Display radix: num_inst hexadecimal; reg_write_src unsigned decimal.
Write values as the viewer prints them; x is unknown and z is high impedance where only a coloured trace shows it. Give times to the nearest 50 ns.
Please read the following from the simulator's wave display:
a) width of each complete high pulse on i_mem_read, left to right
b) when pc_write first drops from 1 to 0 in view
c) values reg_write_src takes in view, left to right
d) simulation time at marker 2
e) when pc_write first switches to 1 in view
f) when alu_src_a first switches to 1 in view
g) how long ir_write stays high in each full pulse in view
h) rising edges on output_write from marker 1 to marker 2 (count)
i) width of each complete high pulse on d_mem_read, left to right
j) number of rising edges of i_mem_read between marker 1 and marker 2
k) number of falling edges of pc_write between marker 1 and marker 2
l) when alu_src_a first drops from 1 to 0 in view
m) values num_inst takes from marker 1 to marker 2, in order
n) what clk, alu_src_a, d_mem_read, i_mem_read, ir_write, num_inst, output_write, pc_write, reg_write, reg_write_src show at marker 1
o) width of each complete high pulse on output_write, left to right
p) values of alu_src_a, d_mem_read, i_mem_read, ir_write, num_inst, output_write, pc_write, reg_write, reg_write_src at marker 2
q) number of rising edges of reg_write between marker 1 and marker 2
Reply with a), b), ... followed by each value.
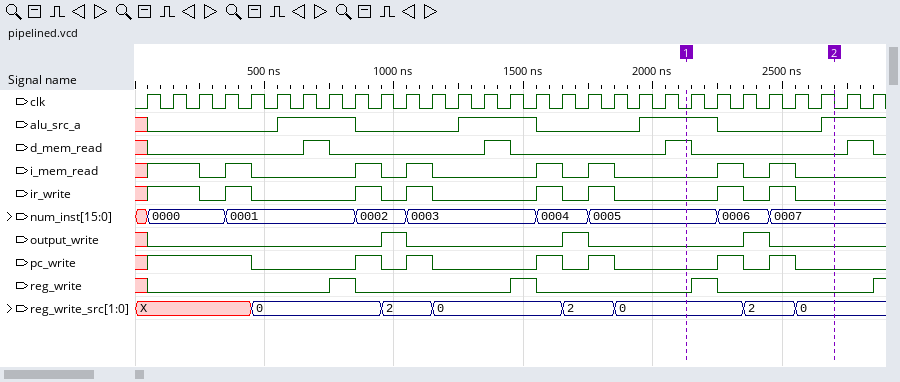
a) 100 ns, 100 ns, 100 ns, 100 ns, 100 ns, 100 ns, 100 ns
b) 450 ns
c) X, 0, 2, 0, 2, 0, 2, 0
d) 2700 ns
e) 50 ns
f) 550 ns
g) 100 ns, 100 ns, 100 ns, 100 ns, 100 ns, 100 ns, 100 ns
h) 1
i) 100 ns, 100 ns, 100 ns, 100 ns
j) 2
k) 2
l) 850 ns
m) 0005, 0006, 0007
n) clk=0, alu_src_a=1, d_mem_read=1, i_mem_read=0, ir_write=0, num_inst=0005, output_write=0, pc_write=0, reg_write=0, reg_write_src=0
o) 100 ns, 100 ns, 100 ns
p) alu_src_a=1, d_mem_read=0, i_mem_read=0, ir_write=0, num_inst=0007, output_write=0, pc_write=0, reg_write=0, reg_write_src=0
q) 1
